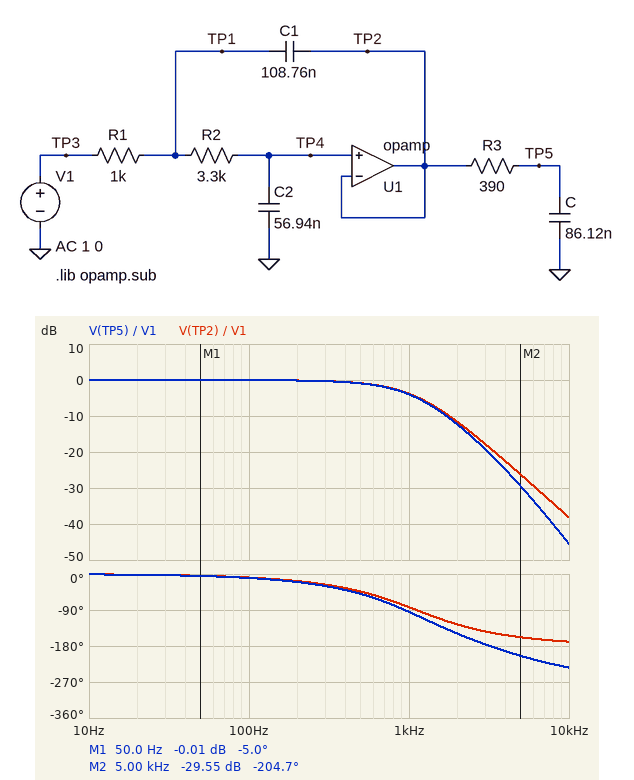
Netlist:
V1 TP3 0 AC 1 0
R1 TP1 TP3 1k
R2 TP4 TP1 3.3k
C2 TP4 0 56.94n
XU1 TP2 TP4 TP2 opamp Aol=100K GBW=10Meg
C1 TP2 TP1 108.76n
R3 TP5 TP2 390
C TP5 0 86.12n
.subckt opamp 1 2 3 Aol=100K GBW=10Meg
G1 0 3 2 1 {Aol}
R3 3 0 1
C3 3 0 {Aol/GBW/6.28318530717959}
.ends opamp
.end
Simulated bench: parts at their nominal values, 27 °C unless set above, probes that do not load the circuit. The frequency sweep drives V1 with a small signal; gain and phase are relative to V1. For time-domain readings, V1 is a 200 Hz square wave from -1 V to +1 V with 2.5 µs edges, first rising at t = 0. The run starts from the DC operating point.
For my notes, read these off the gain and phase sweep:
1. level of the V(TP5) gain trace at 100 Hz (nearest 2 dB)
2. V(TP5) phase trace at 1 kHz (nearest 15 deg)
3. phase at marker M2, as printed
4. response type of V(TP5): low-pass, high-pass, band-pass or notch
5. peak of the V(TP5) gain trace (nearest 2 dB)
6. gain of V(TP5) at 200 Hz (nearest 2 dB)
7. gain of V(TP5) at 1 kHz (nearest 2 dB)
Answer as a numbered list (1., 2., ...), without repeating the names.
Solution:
1. 0 dB
2. -90 deg
3. -204.7 deg
4. low-pass
5. 0 dB
6. 0 dB
7. -4 dB
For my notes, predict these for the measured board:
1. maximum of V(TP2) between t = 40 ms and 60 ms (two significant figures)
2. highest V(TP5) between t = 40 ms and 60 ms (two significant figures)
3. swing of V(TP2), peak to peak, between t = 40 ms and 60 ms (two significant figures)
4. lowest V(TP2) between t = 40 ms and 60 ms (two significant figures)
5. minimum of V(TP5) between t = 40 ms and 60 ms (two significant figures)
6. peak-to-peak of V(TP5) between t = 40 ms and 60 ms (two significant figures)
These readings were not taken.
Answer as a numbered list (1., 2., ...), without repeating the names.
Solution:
1. 1.0 V
2. 1.0 V
3. 2.0 V
4. -1.0 V
5. -1.0 V
6. 2.0 V
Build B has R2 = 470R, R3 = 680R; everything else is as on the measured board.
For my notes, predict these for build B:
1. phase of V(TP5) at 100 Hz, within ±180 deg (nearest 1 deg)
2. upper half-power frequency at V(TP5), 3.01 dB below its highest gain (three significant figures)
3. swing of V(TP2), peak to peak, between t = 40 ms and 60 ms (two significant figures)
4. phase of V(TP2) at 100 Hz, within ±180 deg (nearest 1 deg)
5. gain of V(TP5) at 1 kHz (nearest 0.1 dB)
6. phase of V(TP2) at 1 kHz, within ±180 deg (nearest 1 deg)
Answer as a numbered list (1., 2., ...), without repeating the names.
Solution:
1. -5 deg
2. 1.90 kHz
3. 2.1 V
4. -3 deg
5. -0.8 dB
6. -31 deg
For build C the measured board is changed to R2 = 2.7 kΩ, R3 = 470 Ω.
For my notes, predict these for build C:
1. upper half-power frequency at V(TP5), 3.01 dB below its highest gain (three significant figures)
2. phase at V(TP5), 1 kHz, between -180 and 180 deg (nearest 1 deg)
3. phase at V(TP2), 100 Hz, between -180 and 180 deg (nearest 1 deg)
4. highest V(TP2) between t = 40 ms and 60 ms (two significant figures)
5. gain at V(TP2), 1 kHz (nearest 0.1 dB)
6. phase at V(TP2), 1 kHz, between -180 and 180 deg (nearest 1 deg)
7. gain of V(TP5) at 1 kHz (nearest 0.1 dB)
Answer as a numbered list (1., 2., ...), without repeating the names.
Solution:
1. 1.00 kHz
2. -90 deg
3. -8 deg
4. 1.0 V
5. -2.7 dB
6. -76 deg
7. -3.0 dB
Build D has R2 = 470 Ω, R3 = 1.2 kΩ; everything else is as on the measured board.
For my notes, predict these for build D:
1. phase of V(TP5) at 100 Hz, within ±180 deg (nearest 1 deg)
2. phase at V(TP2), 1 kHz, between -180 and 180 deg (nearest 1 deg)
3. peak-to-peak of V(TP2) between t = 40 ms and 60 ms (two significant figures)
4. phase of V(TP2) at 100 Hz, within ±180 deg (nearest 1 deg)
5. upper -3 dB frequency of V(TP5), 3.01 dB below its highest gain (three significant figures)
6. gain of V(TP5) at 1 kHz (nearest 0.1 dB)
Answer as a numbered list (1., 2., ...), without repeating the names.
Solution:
1. -7 deg
2. -31 deg
3. 2.1 V
4. -3 deg
5. 1.35 kHz
6. -1.8 dB
